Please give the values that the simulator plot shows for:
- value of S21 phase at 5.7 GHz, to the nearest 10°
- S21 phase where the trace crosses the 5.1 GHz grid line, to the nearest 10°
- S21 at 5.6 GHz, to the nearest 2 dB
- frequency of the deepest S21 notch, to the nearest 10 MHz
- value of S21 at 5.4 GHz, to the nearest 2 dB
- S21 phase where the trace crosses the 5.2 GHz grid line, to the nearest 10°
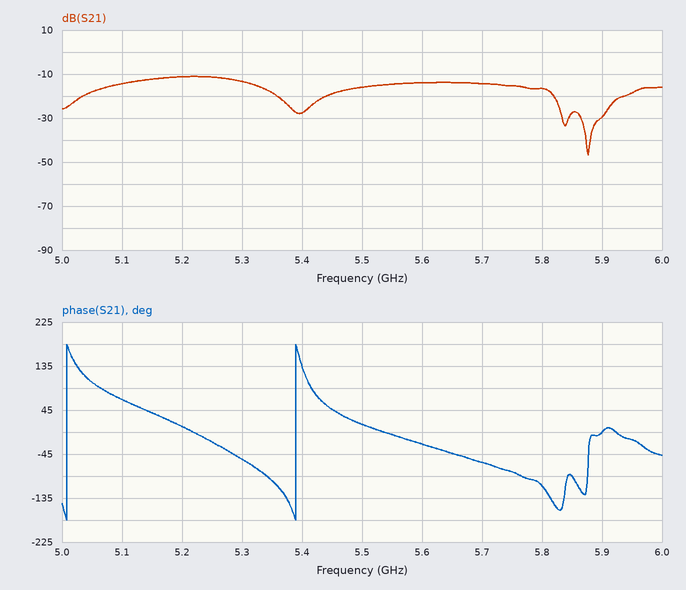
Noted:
-60°
70°
-14 dB
5.88 GHz
-28 dB
10°
